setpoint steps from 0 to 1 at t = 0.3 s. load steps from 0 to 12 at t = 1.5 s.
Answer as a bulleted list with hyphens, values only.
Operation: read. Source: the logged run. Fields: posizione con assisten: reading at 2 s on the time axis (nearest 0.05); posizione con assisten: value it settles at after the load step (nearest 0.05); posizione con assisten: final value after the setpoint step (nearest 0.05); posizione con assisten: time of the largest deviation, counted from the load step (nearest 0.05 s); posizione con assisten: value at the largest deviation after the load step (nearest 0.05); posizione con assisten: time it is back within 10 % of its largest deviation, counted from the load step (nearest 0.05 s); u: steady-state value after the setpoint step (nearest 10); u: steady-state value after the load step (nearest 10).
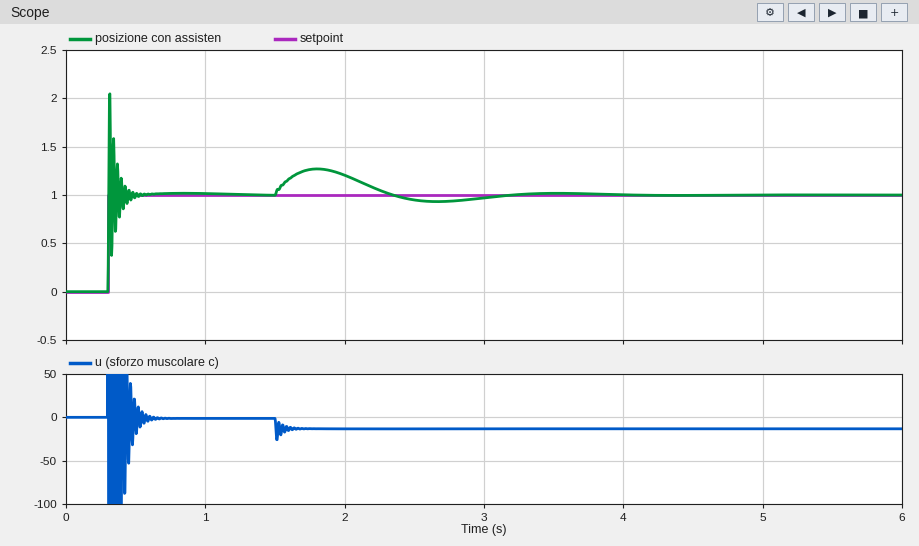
- 1.20
- 1.00
- 1.00
- 0.30 s
- 1.25
- 1.50 s
- 0
- -10
